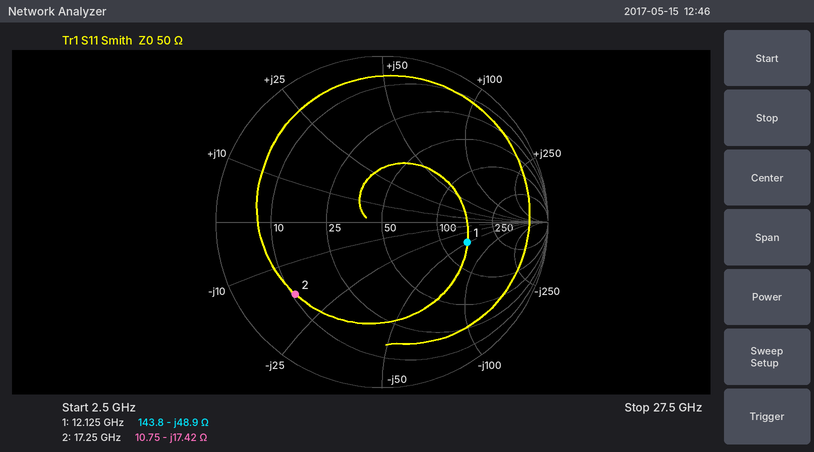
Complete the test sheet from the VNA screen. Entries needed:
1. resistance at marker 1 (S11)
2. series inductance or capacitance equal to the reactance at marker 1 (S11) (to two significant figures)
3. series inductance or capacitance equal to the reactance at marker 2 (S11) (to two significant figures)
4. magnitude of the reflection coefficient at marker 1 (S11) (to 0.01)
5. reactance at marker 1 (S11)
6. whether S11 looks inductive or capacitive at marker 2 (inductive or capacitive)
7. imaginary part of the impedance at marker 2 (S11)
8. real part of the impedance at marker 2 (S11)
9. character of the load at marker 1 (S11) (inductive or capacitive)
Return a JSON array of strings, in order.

["143.8 Ω", "270 fF", "530 fF", "0.53", "-48.9 Ω", "capacitive", "-17.42 Ω", "10.75 Ω", "capacitive"]
